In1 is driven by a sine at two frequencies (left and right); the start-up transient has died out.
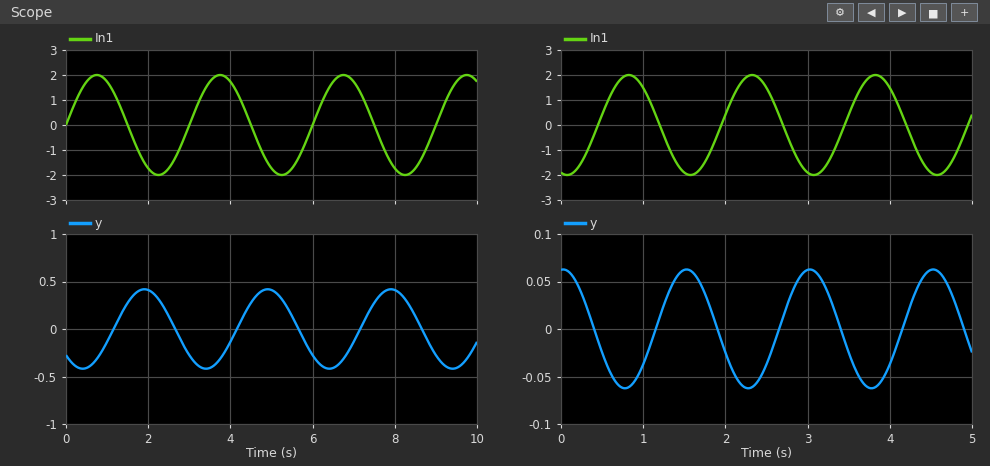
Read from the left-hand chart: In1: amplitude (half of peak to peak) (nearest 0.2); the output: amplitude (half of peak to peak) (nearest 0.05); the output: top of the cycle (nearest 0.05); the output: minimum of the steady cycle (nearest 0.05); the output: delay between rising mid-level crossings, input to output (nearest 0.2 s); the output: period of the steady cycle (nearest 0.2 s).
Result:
2.0
0.40
0.40
-0.40
1.2 s
3.0 s
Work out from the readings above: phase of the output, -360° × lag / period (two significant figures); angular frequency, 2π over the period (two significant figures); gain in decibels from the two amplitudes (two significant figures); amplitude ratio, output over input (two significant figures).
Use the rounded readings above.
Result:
-140°
2.1 rad/s
-14 dB
0.20
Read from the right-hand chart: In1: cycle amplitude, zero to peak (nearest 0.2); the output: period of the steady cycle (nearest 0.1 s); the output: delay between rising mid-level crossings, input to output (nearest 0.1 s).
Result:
2.0
1.5 s
0.7 s
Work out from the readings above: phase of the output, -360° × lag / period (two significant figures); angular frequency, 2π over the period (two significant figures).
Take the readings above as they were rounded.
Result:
-170°
4.2 rad/s
